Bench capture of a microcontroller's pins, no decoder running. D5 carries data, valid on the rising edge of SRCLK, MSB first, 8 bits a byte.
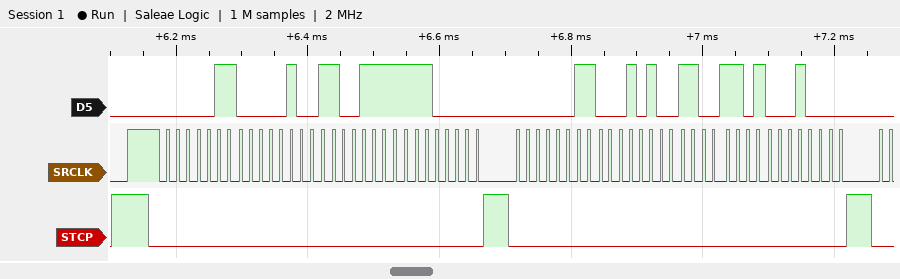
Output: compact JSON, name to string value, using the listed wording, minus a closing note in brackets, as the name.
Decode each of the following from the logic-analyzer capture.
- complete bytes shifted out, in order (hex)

{"complete bytes shifted out, in order": "03 04 CF E0 03 14 CD 10"}
